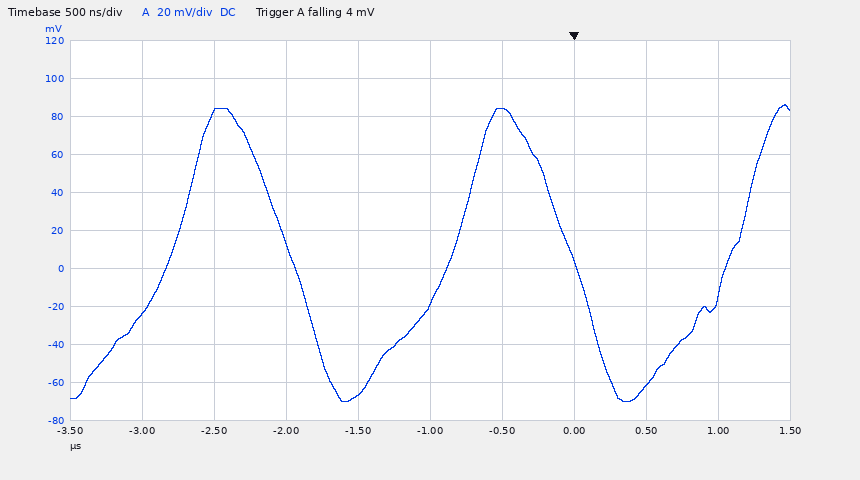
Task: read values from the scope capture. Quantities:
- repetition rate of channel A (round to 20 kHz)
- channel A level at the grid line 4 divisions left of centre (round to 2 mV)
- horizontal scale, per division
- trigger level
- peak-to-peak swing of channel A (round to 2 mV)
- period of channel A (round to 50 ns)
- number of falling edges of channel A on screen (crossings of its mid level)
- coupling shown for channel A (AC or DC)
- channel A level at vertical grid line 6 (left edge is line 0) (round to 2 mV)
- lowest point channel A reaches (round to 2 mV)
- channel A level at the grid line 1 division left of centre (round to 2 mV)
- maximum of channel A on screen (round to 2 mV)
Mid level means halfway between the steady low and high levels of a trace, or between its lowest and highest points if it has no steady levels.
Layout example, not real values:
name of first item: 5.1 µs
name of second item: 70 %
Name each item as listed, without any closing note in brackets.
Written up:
repetition rate of channel A: 520 kHz
channel A level at the grid line 4 divisions left of centre: -24 mV
horizontal scale, per division: 500 ns
trigger level: 4 mV
peak-to-peak swing of channel A: 156 mV
period of channel A: 1.95 µs
number of falling edges of channel A on screen: 2
coupling shown for channel A: DC
channel A level at vertical grid line 6 (left edge is line 0): 84 mV
lowest point channel A reaches: -70 mV
channel A level at the grid line 1 division left of centre: -66 mV
maximum of channel A on screen: 86 mV
